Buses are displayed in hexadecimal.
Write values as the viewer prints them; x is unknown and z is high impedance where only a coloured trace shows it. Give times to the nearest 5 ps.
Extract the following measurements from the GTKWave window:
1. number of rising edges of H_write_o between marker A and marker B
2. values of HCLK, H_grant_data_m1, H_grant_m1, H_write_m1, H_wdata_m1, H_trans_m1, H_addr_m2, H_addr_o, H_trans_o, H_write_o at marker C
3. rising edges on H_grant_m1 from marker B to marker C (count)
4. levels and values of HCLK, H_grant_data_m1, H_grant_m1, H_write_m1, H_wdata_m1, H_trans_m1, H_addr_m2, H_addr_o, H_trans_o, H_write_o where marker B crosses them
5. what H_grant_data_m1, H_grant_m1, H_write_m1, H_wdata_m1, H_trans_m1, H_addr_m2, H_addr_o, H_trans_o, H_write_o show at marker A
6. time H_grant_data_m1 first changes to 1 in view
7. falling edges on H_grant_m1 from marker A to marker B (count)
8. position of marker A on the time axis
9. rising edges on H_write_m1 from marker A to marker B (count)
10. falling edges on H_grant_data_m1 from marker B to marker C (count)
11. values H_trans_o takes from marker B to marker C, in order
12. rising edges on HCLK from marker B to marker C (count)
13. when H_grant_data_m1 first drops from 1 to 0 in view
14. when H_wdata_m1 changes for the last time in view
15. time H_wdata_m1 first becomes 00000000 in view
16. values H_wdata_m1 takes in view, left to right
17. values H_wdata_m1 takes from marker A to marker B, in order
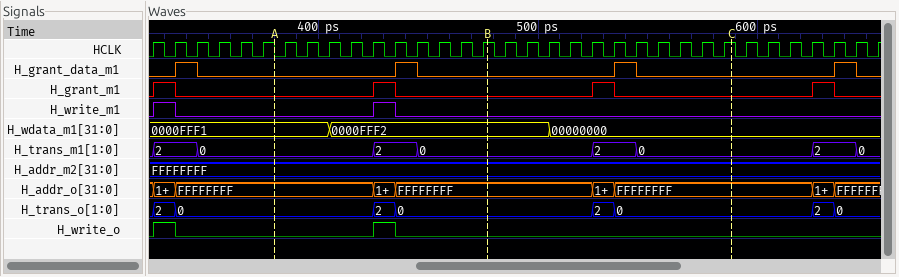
1
HCLK=1, H_grant_data_m1=0, H_grant_m1=0, H_write_m1=0, H_wdata_m1=00000000, H_trans_m1=0, H_addr_m2=FFFFFFFF, H_addr_o=FFFFFFFF, H_trans_o=0, H_write_o=0
1
HCLK=1, H_grant_data_m1=0, H_grant_m1=0, H_write_m1=0, H_wdata_m1=0000FFF2, H_trans_m1=0, H_addr_m2=FFFFFFFF, H_addr_o=FFFFFFFF, H_trans_o=0, H_write_o=0
H_grant_data_m1=0, H_grant_m1=0, H_write_m1=0, H_wdata_m1=0000FFF1, H_trans_m1=0, H_addr_m2=FFFFFFFF, H_addr_o=FFFFFFFF, H_trans_o=0, H_write_o=0
335 ps
1
380 ps
1
1
0, 2, 0
11
345 ps
505 ps
505 ps
0000FFF1, 0000FFF2, 00000000
0000FFF1, 0000FFF2
